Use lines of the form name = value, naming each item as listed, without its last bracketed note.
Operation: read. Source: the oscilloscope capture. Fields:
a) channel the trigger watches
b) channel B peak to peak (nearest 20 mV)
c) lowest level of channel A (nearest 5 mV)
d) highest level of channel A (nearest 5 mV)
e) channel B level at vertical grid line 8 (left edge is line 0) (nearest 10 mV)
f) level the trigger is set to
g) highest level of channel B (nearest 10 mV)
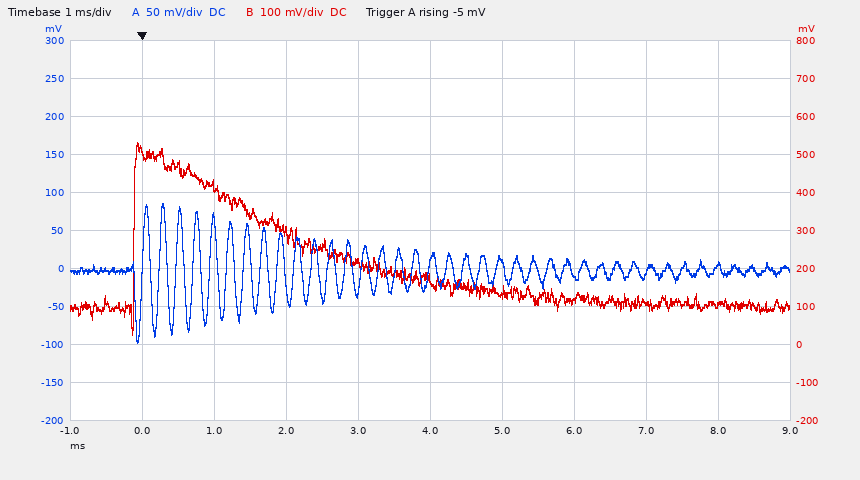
channel the trigger watches = channel A
channel B peak to peak = 500 mV
lowest level of channel A = -95 mV
highest level of channel A = 85 mV
channel B level at vertical grid line 8 (left edge is line 0) = 110 mV
level the trigger is set to = -5 mV
highest level of channel B = 530 mV
